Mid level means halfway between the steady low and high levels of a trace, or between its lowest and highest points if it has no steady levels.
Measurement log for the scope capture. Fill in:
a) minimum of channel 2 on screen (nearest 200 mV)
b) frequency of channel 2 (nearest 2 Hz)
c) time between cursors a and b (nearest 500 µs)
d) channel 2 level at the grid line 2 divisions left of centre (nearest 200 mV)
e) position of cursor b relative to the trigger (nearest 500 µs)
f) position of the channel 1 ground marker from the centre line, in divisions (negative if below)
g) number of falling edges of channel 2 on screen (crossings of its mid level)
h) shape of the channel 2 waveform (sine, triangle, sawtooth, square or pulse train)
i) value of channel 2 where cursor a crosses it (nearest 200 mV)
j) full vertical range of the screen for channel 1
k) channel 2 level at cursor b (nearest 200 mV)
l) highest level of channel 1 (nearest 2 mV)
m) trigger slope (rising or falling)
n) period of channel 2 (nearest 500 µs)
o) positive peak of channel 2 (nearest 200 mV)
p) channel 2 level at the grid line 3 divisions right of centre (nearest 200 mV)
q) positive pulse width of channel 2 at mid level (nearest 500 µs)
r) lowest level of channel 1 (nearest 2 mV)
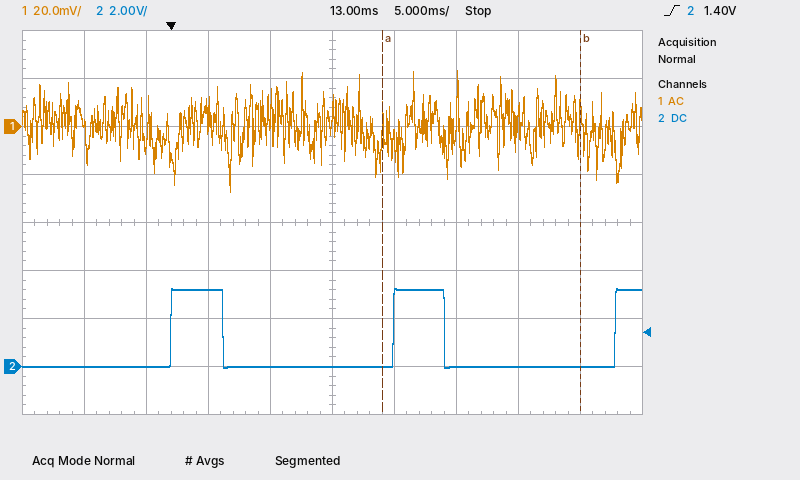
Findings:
0.0 V
56 Hz
16.0 ms
3.2 V
+33.0 ms
+2.0 div
2
pulse train
0.0 V
160 mV
0.0 V
24 mV
rising
18.0 ms
3.2 V
0.0 V
4.0 ms
-28 mV
